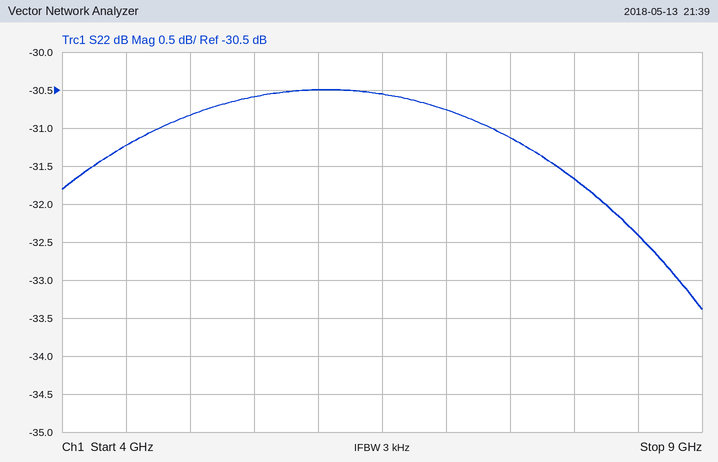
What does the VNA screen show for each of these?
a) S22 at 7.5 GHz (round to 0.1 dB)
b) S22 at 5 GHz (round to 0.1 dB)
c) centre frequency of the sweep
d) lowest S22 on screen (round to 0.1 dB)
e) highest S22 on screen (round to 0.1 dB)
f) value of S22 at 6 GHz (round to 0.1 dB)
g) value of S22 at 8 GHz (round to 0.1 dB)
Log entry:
-31.1 dB
-30.8 dB
6.5 GHz
-33.4 dB
-30.5 dB
-30.5 dB
-31.7 dB
